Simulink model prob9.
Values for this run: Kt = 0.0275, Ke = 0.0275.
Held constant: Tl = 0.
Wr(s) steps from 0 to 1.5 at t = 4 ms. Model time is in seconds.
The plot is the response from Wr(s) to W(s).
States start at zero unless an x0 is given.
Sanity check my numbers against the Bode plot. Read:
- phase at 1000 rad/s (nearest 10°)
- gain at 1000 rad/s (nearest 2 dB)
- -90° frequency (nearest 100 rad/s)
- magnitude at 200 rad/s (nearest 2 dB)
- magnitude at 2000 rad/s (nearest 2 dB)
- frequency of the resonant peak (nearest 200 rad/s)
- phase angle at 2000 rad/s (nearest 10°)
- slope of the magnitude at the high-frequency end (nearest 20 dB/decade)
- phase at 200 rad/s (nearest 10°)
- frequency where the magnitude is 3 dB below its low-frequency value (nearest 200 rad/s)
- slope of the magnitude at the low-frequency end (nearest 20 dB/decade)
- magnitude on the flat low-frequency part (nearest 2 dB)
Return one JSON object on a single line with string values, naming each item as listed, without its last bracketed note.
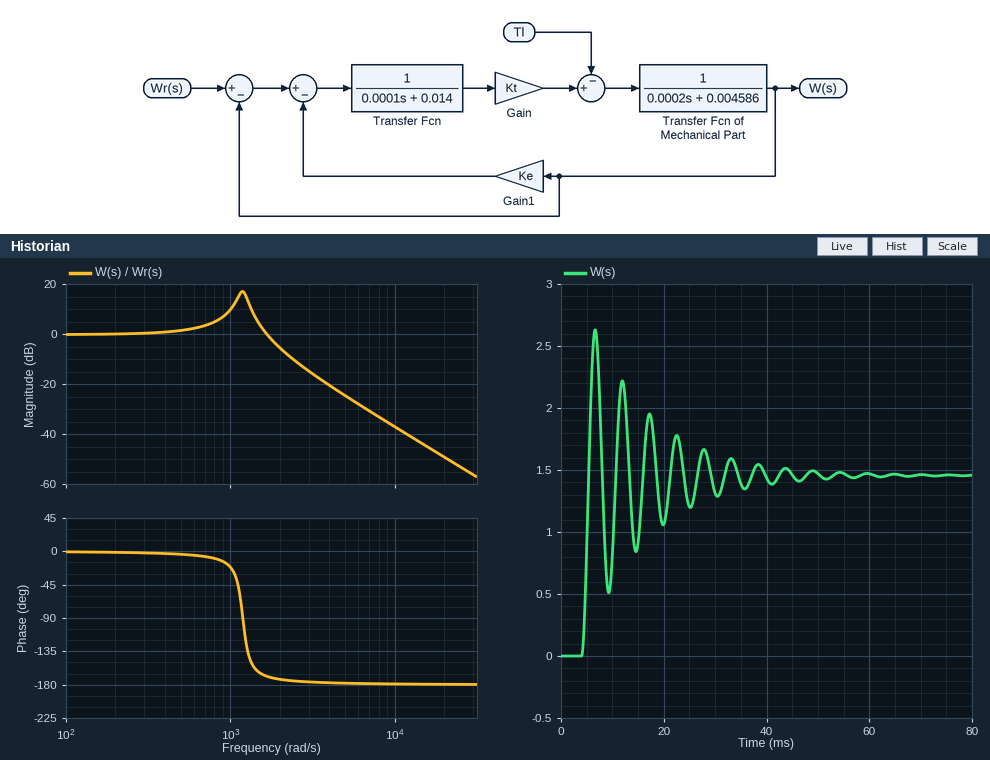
{"phase at 1000 rad/s": "-20°", "gain at 1000 rad/s": "10 dB", "-90° frequency": "1200 rad/s", "magnitude at 200 rad/s": "0 dB", "magnitude at 2000 rad/s": "-6 dB", "frequency of the resonant peak": "1200 rad/s", "phase angle at 2000 rad/s": "-170°", "slope of the magnitude at the high-frequency end": "-40 dB/decade", "phase at 200 rad/s": "0°", "frequency where the magnitude is 3 dB below its low-frequency value": "1800 rad/s", "slope of the magnitude at the low-frequency end": "0 dB/decade", "magnitude on the flat low-frequency part": "0 dB"}
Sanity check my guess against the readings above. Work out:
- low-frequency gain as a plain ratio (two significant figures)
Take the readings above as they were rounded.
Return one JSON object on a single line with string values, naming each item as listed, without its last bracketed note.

{"low-frequency gain as a plain ratio": "1.0"}
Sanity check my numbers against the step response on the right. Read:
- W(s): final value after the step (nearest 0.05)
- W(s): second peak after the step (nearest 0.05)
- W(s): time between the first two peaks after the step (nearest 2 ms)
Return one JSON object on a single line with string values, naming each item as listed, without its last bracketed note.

{"W(s): final value after the step": "1.45", "W(s): second peak after the step": "2.20", "W(s): time between the first two peaks after the step": "6 ms"}
